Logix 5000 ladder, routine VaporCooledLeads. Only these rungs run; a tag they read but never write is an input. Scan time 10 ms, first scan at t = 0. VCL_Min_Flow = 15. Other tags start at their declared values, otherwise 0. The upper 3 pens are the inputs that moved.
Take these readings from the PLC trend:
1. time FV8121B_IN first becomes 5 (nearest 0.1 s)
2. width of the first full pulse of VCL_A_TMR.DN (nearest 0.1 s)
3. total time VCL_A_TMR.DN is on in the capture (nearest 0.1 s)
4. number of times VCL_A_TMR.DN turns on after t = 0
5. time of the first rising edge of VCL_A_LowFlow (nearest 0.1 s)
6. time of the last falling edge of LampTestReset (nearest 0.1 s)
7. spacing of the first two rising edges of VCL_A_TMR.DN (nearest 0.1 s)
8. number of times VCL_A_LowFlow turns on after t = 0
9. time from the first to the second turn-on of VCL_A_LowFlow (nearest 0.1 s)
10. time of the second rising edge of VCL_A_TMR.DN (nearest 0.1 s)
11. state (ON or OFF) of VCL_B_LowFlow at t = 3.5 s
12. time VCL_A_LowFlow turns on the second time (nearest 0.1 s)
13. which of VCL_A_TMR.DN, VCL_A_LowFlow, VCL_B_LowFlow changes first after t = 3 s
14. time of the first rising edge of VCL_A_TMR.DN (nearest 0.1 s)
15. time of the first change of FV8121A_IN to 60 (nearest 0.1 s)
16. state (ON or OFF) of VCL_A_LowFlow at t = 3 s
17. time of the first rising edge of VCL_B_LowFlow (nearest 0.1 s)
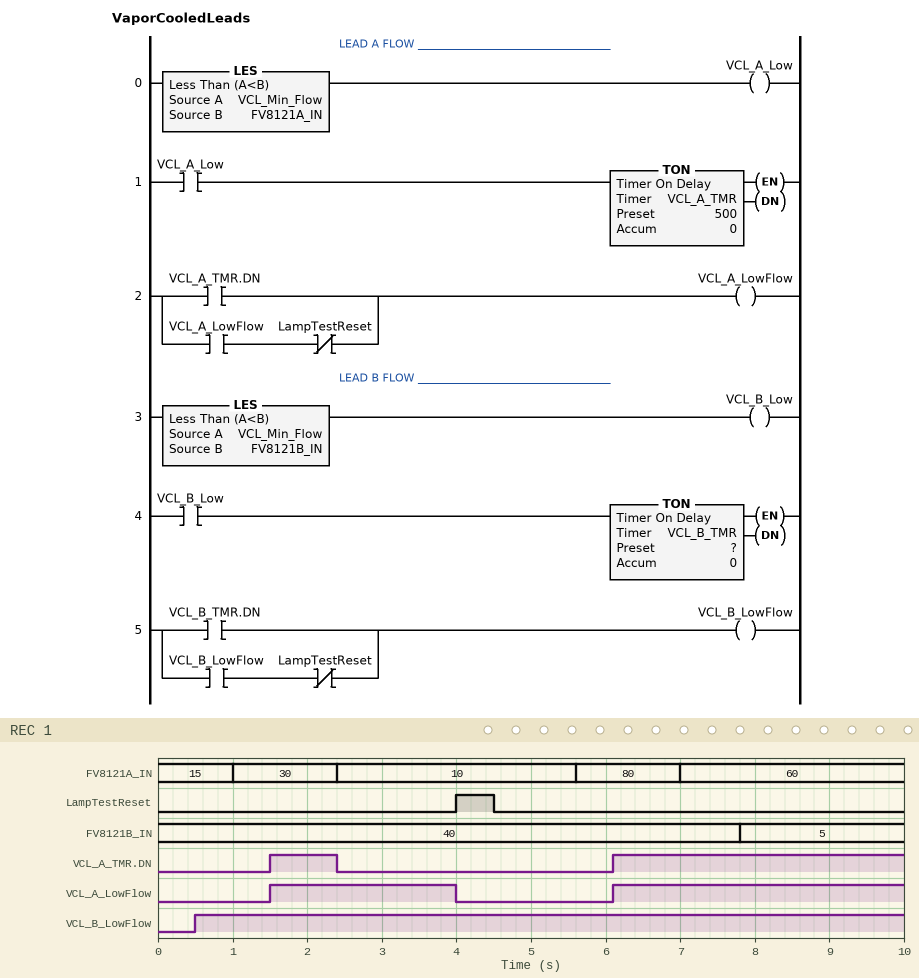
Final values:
7.8 s
0.9 s
4.8 s
2
1.5 s
4.5 s
4.6 s
2
4.6 s
6.1 s
ON
6.1 s
VCL_A_LowFlow
1.5 s
7.0 s
ON
0.5 s
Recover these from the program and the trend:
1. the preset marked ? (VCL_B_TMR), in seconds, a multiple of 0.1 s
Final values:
0.5 s
